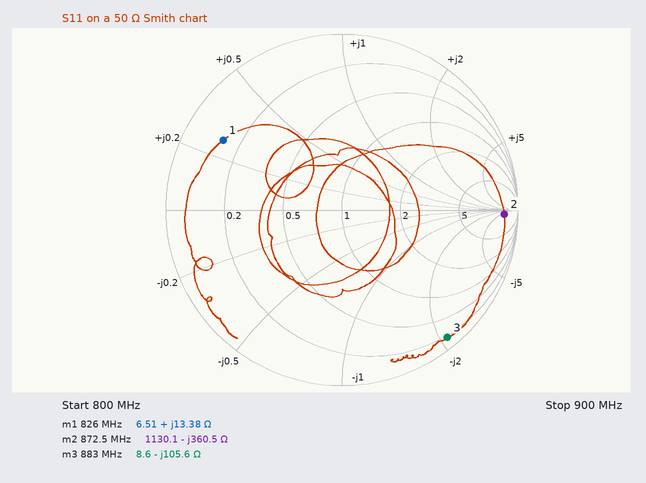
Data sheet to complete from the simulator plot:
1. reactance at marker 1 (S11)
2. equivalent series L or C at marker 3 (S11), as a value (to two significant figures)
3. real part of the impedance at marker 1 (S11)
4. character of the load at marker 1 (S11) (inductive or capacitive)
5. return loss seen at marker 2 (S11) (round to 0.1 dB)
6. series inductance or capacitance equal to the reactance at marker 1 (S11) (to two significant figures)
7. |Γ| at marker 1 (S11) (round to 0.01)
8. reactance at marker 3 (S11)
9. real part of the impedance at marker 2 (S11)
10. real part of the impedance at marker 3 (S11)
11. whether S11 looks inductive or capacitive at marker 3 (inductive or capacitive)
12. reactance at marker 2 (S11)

+13.38 Ω
1.7 pF
6.51 Ω
inductive
0.7 dB
2.6 nH
0.78
-105.6 Ω
1130.1 Ω
8.6 Ω
capacitive
-360.5 Ω
